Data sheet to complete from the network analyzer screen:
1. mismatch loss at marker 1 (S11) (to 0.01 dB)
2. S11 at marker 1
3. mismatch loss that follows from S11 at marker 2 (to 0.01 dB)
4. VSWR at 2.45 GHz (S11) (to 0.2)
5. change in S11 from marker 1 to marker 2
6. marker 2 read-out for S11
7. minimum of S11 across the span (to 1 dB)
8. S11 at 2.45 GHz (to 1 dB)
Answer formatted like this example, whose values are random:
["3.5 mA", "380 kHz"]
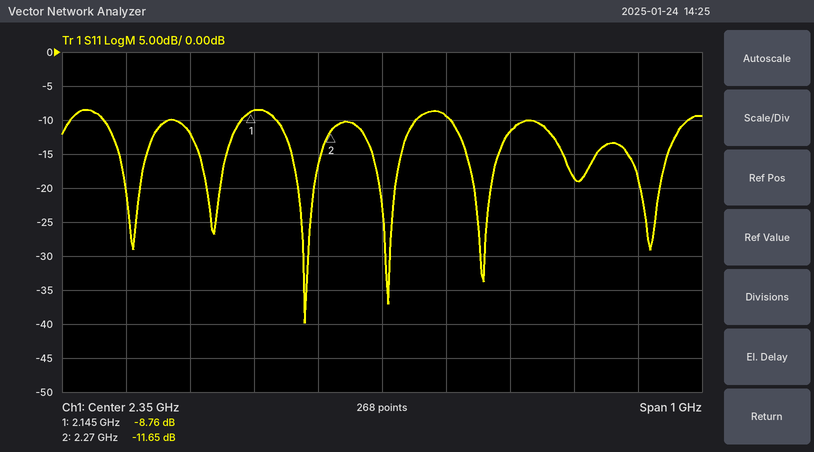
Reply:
["0.62 dB", "-8.76 dB", "0.31 dB", "2.0", "-2.89 dB", "-11.65 dB", "-40 dB", "-9 dB"]
